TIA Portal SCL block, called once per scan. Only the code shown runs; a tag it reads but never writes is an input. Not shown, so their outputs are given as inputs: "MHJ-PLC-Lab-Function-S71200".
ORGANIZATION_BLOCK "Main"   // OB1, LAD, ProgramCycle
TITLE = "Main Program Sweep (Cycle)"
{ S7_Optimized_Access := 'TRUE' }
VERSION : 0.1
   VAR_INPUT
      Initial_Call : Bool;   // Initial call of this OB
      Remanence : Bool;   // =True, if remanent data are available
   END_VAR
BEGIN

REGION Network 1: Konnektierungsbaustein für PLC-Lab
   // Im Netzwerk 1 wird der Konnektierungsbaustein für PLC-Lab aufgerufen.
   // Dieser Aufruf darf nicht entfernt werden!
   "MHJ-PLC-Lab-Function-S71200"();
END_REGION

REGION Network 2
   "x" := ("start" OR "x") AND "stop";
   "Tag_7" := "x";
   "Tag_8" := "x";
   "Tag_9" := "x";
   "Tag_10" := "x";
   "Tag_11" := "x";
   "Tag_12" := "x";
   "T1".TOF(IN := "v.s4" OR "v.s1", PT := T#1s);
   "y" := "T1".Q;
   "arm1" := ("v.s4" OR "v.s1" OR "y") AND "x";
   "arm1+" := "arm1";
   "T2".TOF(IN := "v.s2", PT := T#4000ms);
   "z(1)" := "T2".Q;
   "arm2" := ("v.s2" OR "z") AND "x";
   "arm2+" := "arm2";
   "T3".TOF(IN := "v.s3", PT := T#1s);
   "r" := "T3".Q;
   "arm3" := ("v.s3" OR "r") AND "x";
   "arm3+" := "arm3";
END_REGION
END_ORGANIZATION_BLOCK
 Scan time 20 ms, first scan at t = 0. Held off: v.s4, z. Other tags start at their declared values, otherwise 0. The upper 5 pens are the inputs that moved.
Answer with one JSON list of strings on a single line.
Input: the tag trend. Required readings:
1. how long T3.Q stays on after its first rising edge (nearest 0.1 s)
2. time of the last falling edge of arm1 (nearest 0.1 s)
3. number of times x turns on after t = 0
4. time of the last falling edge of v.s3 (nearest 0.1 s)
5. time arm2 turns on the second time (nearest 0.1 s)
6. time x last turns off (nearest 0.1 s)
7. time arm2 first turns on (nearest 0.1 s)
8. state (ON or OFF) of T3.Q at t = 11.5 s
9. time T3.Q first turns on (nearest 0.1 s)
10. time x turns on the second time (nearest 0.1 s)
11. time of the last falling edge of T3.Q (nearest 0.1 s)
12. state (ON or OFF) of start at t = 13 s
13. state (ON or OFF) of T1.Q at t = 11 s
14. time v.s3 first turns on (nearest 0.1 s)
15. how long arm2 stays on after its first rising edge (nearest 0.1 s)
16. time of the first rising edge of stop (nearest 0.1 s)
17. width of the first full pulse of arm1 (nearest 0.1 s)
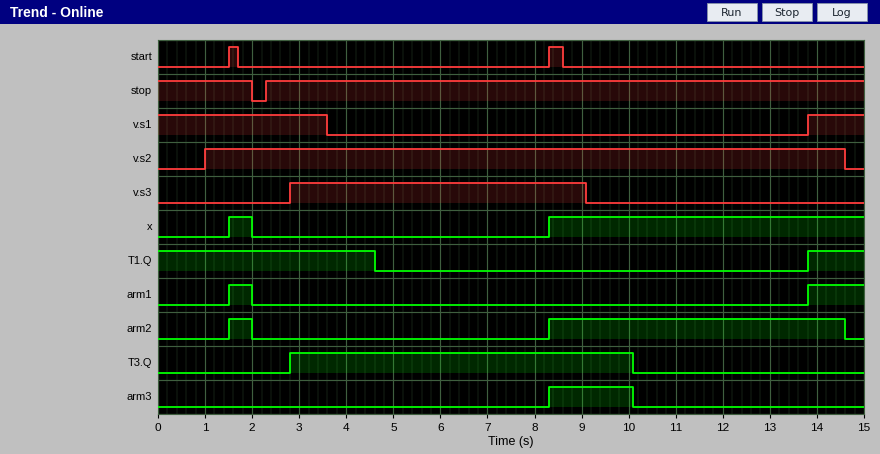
["7.3 s", "2.0 s", "2", "9.1 s", "8.3 s", "2.0 s", "1.5 s", "OFF", "2.8 s", "8.3 s", "10.1 s", "OFF", "OFF", "2.8 s", "0.5 s", "2.3 s", "0.5 s"]
